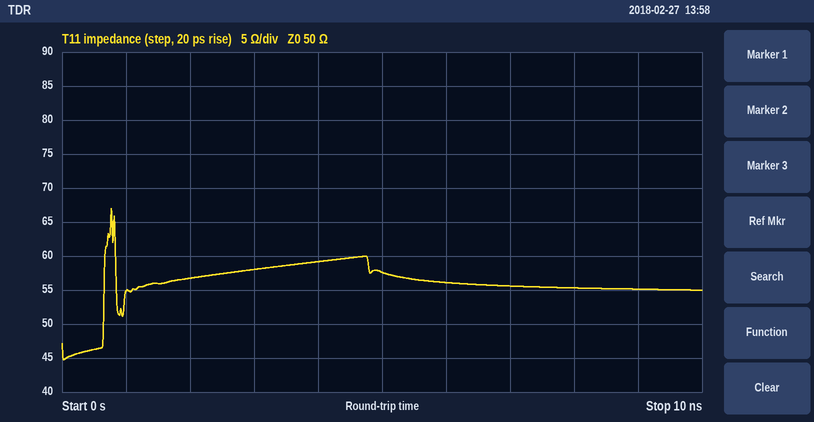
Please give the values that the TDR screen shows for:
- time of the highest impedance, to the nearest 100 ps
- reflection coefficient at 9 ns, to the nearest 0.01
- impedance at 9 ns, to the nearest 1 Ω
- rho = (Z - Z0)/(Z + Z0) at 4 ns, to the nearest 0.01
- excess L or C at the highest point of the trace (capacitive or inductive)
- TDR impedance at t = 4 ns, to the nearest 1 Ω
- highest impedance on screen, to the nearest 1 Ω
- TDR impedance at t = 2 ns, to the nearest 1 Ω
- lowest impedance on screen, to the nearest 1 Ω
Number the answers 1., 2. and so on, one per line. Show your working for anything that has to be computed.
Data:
1. 800 ps
2. (55 − 50)/(55 + 50) ≈ +0.05
3. 55 Ω
4. (59 − 50)/(59 + 50) ≈ +0.08
5. inductive
6. 59 Ω
7. 67 Ω
8. 57 Ω
9. 45 Ω
